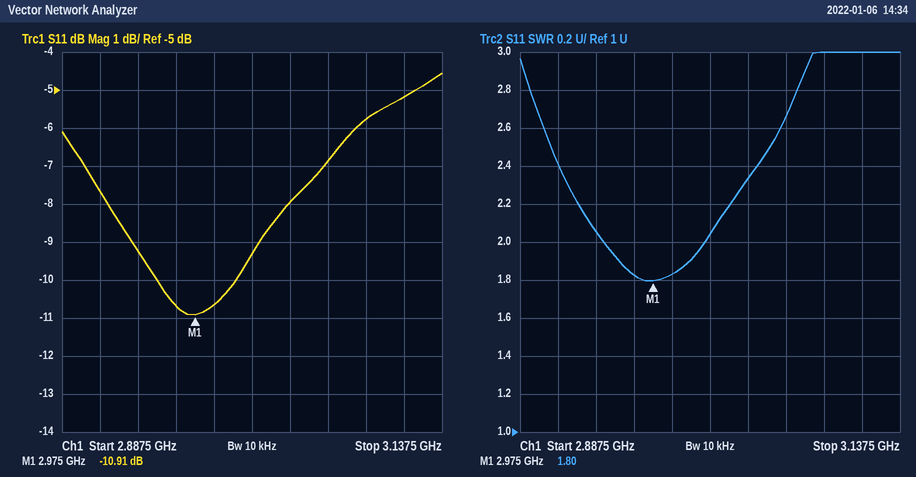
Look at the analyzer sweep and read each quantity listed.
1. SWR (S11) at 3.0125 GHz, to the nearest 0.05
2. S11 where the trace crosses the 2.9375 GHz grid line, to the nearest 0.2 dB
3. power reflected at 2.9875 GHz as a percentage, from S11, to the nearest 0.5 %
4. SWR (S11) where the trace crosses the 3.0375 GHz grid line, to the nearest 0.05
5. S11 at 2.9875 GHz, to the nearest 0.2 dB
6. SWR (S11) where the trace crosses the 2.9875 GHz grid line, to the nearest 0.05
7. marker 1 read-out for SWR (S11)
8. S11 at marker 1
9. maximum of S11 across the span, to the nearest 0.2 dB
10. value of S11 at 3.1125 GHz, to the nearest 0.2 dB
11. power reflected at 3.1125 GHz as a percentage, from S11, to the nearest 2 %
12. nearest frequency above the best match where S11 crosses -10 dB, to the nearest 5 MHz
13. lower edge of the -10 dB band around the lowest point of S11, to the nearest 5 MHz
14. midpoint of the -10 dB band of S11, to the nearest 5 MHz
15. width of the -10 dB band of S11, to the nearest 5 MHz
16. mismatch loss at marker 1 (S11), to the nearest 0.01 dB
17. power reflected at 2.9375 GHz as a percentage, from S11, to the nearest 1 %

2.05
-9.2 dB
8.5 %
2.35
-10.6 dB
1.85
1.80
-10.91 dB
-4.6 dB
-5.2 dB
30 %
3.000 GHz
2.950 GHz
2.975 GHz
50 MHz
0.37 dB
12 %
